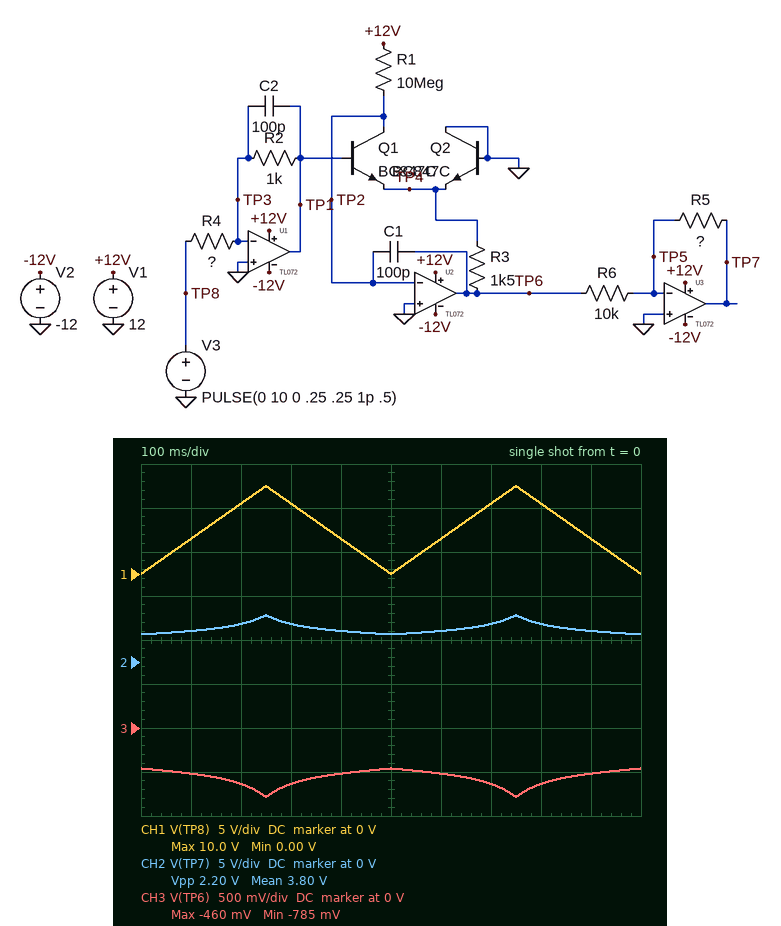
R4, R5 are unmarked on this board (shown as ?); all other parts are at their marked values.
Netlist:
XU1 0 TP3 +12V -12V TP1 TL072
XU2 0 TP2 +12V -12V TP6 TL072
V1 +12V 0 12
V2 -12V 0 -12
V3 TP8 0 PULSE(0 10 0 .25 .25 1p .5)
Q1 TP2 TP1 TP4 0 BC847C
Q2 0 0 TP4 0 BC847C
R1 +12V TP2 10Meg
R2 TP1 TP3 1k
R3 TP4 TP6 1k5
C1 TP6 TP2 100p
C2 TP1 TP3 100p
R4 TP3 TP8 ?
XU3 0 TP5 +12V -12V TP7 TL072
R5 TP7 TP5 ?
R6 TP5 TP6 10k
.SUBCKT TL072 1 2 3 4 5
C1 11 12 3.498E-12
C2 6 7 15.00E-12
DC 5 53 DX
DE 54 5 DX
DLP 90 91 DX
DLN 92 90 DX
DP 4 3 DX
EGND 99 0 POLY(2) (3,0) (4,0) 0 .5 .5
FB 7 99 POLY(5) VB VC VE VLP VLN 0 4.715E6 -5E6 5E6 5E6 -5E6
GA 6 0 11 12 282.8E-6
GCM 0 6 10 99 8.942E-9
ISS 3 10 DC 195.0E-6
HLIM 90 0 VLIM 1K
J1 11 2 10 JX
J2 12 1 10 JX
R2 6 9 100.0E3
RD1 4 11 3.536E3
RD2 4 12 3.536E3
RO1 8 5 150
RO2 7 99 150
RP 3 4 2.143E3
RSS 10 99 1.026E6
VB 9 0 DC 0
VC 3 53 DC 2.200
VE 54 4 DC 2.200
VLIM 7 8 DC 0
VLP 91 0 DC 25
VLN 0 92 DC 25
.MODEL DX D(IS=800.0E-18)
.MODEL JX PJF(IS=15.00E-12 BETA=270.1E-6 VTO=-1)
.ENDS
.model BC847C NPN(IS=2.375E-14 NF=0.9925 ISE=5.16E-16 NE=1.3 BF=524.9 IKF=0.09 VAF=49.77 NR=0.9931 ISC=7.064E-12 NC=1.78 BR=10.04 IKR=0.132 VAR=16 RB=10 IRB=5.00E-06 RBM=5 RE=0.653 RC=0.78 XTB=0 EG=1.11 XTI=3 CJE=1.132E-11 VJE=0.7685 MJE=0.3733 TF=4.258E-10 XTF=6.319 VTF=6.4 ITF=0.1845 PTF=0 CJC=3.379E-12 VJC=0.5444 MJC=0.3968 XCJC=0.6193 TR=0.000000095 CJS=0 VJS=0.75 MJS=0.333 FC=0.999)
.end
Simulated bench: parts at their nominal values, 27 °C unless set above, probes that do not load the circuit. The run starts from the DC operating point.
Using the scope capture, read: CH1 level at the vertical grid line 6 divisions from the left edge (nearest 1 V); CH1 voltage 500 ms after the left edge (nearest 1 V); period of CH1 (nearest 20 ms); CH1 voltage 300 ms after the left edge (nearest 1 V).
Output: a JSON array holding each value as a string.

["4 V", "0 V", "500 ms", "8 V"]
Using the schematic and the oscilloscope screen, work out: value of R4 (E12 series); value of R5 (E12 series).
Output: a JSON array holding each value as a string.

["82 kΩ", "68 kΩ"]
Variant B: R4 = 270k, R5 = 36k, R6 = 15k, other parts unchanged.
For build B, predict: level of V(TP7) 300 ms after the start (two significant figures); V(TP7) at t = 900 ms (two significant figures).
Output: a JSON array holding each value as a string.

["1.2 V", "1.1 V"]
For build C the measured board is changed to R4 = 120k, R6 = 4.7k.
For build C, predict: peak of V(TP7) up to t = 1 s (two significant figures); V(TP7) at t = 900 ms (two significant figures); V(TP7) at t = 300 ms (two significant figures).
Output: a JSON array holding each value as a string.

["8.5 V", "7.2 V", "7.9 V"]
